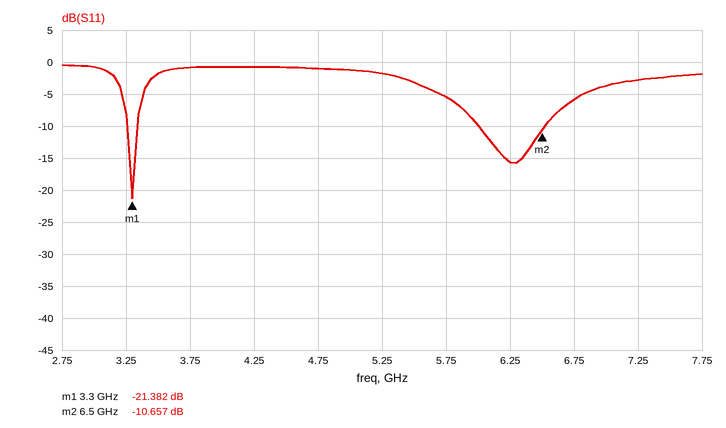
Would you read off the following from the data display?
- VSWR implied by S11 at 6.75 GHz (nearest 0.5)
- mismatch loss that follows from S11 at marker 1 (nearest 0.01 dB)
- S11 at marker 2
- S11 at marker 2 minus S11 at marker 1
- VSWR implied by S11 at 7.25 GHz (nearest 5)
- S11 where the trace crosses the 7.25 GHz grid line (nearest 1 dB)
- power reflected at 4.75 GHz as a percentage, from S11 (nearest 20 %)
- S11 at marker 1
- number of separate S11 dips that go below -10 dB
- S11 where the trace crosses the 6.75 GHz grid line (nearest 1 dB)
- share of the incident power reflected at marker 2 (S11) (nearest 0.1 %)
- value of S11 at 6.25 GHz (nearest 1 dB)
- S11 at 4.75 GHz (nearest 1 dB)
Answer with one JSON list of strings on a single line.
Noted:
["3.0", "0.03 dB", "-10.657 dB", "10.725 dB", "5", "-3 dB", "80 %", "-21.382 dB", "2", "-6 dB", "8.6 %", "-16 dB", "-1 dB"]
